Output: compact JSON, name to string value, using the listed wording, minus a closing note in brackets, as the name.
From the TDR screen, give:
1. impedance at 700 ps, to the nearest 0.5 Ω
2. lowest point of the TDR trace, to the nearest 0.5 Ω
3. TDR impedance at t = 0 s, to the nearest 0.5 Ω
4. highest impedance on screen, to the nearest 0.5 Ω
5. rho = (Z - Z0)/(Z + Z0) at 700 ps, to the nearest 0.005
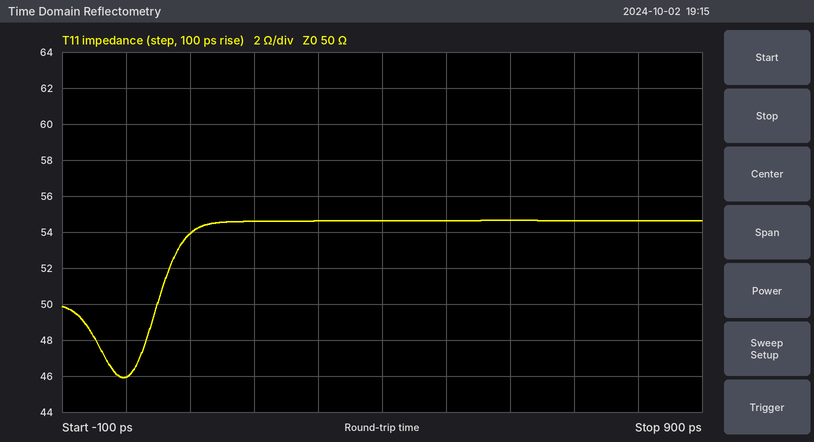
{"impedance at 700 ps, to the nearest 0.5 Ω": "54.5 Ω", "lowest point of the TDR trace, to the nearest 0.5 Ω": "46.0 Ω", "TDR impedance at t = 0 s, to the nearest 0.5 Ω": "46.0 Ω", "highest impedance on screen, to the nearest 0.5 Ω": "54.5 Ω", "rho = (Z - Z0)/(Z + Z0) at 700 ps, to the nearest 0.005": "+0.045"}
